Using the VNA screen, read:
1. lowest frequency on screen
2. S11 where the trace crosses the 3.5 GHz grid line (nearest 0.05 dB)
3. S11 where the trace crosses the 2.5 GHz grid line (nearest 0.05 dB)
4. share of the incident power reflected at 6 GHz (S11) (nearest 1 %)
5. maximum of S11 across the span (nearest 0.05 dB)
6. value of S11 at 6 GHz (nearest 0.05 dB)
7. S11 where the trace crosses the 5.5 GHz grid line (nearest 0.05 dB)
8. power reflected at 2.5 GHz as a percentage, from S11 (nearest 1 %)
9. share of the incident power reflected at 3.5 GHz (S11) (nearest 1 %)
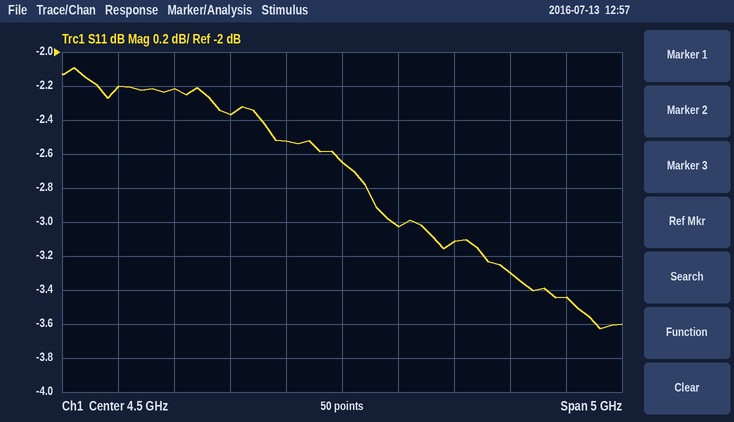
2 GHz
-2.35 dB
-2.20 dB
47 %
-2.10 dB
-3.30 dB
-3.10 dB
60 %
58 %
